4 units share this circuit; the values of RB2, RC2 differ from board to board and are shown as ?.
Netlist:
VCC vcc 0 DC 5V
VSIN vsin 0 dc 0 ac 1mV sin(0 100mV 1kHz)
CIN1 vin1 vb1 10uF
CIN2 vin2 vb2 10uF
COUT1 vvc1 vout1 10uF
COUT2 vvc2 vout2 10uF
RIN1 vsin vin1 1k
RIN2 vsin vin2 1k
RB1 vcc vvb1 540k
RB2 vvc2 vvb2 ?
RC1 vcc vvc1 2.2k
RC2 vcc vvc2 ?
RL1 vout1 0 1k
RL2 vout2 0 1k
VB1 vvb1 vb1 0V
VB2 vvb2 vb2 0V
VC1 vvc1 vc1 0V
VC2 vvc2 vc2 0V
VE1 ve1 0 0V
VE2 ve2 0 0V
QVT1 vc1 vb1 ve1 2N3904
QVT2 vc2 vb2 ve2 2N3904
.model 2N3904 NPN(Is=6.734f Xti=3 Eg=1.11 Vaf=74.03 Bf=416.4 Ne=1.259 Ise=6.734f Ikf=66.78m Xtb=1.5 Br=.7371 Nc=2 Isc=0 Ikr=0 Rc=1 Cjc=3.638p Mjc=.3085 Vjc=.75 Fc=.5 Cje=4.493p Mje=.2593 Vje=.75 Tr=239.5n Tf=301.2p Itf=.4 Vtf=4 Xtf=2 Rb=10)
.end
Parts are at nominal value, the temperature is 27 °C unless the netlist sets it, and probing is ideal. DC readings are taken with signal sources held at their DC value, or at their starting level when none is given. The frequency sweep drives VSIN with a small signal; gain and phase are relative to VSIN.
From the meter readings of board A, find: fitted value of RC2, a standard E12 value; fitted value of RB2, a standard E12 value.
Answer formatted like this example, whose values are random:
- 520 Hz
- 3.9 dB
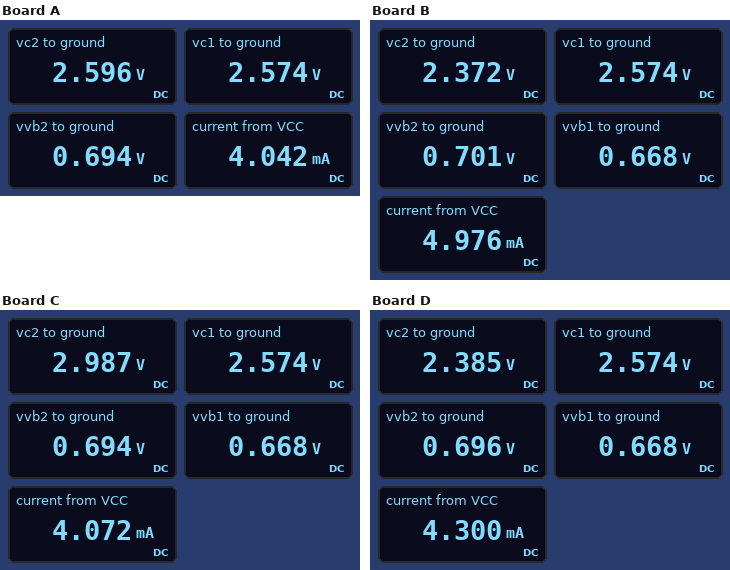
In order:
- 820 Ω
- 100 kΩ
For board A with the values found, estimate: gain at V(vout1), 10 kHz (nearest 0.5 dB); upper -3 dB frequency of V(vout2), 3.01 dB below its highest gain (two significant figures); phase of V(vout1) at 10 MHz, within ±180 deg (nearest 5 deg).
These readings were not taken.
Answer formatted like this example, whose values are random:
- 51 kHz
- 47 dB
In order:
- 27.0 dB
- 2.1 MHz
- 100 deg
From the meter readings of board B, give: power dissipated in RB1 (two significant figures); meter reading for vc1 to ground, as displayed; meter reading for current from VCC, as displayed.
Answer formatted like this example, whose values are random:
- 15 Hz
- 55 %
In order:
- 35 µW
- 2.574 V
- 4.976 mA
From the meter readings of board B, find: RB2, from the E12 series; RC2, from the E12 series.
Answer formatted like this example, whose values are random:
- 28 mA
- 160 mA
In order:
- 68 kΩ
- 680 Ω
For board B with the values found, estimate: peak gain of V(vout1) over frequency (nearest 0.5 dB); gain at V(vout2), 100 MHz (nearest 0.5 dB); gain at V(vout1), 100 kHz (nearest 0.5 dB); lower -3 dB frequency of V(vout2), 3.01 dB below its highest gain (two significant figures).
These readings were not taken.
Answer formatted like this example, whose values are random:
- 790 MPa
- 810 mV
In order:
- 27.0 dB
- -7.0 dB
- 27.0 dB
- 16 Hz
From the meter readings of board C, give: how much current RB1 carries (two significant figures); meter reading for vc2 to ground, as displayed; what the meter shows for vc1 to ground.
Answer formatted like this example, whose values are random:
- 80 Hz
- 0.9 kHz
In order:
- 8.0 µA
- 2.987 V
- 2.574 V
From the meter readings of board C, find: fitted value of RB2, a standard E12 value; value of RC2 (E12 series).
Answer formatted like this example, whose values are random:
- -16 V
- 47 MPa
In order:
- 120 kΩ
- 680 Ω
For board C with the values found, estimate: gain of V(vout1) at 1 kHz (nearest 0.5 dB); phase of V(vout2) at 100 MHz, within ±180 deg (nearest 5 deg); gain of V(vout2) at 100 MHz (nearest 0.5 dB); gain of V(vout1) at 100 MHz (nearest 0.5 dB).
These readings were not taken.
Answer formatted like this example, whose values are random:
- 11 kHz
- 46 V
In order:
- 27.0 dB
- 80 deg
- -6.5 dB
- -6.5 dB
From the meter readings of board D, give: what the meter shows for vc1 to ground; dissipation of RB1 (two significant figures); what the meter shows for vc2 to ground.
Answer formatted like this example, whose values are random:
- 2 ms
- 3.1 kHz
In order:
- 2.574 V
- 35 µW
- 2.385 V
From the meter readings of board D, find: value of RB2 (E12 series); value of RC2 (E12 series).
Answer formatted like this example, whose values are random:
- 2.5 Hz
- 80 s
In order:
- 82 kΩ
- 820 Ω
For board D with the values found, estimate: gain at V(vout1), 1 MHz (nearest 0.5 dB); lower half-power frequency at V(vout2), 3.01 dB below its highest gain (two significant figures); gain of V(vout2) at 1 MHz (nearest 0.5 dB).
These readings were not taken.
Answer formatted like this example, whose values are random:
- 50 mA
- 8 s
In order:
- 26.0 dB
- 15 Hz
- 26.0 dB
